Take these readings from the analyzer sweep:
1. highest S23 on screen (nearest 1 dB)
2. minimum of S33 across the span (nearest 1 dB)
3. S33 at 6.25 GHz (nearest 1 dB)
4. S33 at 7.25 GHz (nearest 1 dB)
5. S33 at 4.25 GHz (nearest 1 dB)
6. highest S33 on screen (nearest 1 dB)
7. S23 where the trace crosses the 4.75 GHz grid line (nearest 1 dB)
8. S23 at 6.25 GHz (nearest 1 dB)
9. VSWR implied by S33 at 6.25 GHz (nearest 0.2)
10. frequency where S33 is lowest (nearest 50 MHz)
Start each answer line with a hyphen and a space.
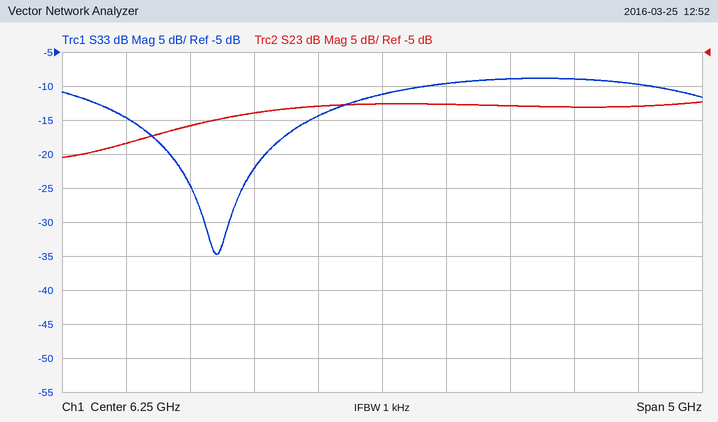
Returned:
- -12 dB
- -35 dB
- -11 dB
- -9 dB
- -15 dB
- -9 dB
- -16 dB
- -13 dB
- 1.8
- 4.95 GHz
